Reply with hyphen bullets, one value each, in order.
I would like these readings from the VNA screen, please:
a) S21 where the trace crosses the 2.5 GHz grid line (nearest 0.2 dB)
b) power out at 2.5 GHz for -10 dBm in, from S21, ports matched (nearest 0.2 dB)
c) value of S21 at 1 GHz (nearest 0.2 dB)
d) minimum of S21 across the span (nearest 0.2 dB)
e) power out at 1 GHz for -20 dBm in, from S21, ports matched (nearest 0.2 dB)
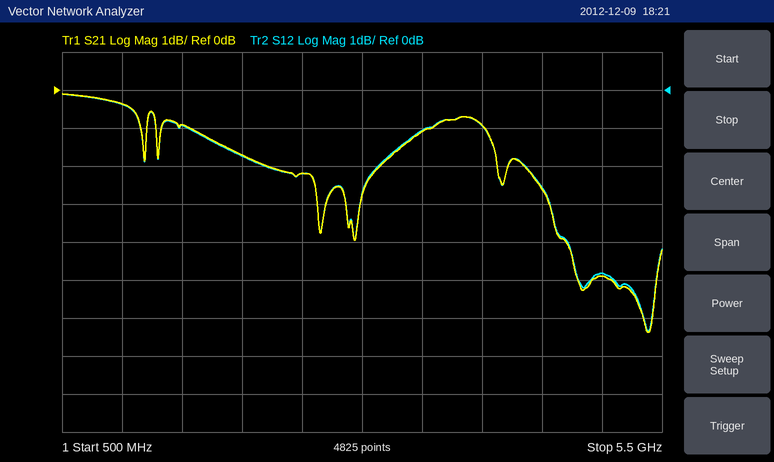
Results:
- -2.2 dB
- -12.2 dBm
- -0.4 dB
- -6.4 dB
- -20.4 dBm
